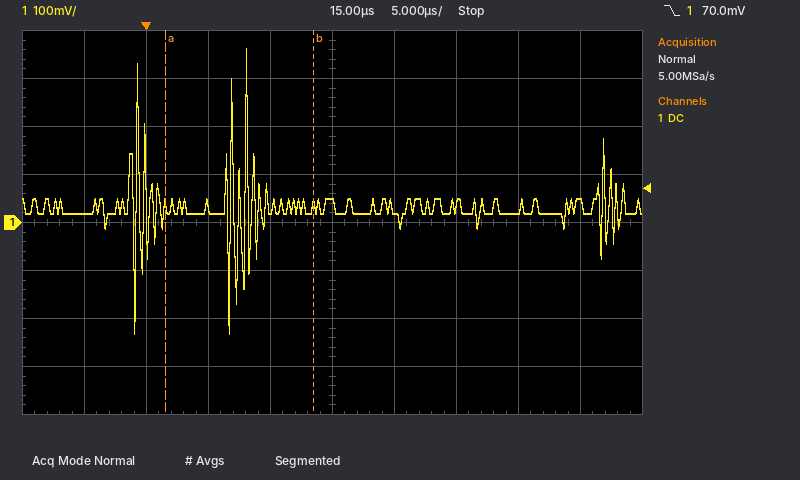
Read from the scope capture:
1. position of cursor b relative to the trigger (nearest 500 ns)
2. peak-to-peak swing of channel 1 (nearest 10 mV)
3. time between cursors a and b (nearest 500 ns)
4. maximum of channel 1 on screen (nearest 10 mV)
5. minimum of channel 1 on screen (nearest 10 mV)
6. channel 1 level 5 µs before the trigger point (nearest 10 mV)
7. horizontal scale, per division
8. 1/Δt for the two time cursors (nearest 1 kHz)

+13.5 µs
590 mV
12.0 µs
360 mV
-230 mV
20 mV
5 µs
83 kHz
